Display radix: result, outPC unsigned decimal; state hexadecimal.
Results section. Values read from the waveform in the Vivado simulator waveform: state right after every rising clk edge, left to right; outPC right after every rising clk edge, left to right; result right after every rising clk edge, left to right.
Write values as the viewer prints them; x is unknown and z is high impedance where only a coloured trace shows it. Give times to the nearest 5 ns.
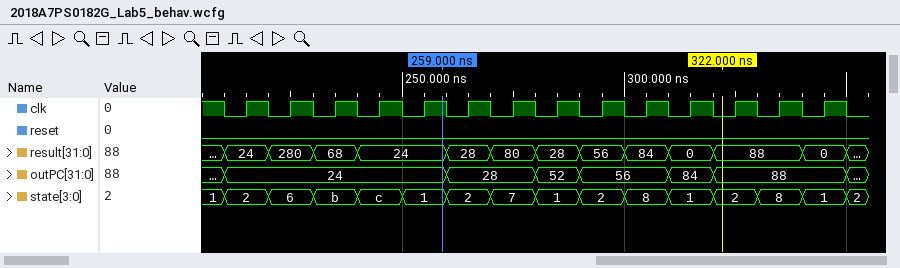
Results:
2, 6, b, c, 1, 2, 7, 1, 2, 8, 1, 2, 8, 1
24, 24, 24, 24, 24, 28, 28, 52, 56, 56, 84, 88, 88, 88
24, 280, 68, 24, 24, 28, 80, 28, 56, 84, 0, 88, 88, 0
